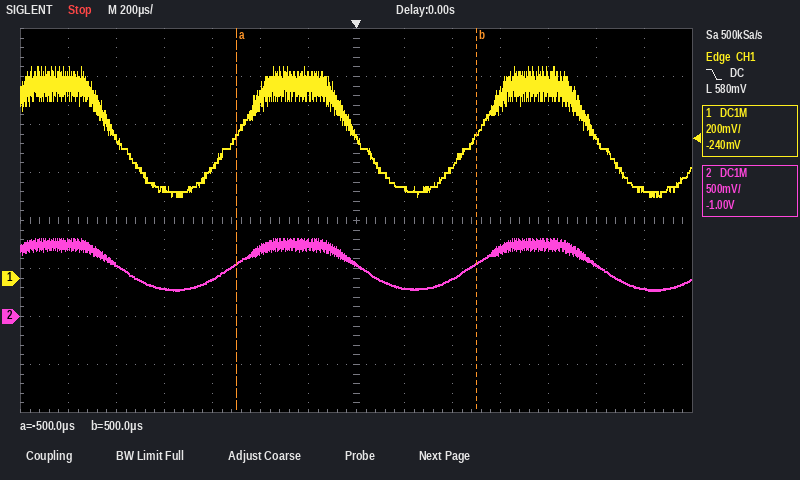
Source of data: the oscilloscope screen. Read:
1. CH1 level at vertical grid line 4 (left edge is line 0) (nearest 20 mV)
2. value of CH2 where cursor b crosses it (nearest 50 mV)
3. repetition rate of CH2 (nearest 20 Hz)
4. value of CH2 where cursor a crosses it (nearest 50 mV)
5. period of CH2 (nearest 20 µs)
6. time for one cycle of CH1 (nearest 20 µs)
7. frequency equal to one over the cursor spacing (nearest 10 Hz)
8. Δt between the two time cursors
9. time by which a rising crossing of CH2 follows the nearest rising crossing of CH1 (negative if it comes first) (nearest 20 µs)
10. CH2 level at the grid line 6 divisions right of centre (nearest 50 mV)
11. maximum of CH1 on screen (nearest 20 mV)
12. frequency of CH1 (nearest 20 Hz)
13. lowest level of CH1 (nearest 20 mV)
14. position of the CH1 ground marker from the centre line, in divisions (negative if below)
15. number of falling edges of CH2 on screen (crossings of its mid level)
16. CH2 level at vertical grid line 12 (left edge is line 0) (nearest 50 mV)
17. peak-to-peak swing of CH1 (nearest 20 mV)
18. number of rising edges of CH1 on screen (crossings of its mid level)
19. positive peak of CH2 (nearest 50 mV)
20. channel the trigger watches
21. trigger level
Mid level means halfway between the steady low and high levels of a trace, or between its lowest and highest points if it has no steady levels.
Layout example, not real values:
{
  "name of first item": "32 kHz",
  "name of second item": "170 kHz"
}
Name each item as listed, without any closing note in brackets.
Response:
{
  "CH1 level at vertical grid line 4 (left edge is line 0)": "460 mV",
  "value of CH2 where cursor b crosses it": "550 mV",
  "repetition rate of CH2": "1.00 kHz",
  "value of CH2 where cursor a crosses it": "550 mV",
  "period of CH2": "1.00 ms",
  "time for one cycle of CH1": "1.00 ms",
  "frequency equal to one over the cursor spacing": "1.00 kHz",
  "Δt between the two time cursors": "1.00 ms",
  "time by which a rising crossing of CH2 follows the nearest rising crossing of CH1 (negative if it comes first)": "-20 µs",
  "CH2 level at the grid line 6 divisions right of centre": "300 mV",
  "maximum of CH1 on screen": "880 mV",
  "frequency of CH1": "1.00 kHz",
  "lowest level of CH1": "340 mV",
  "position of the CH1 ground marker from the centre line, in divisions": "-1.2 div",
  "number of falling edges of CH2 on screen": "3",
  "CH2 level at vertical grid line 12 (left edge is line 0)": "550 mV",
  "peak-to-peak swing of CH1": "540 mV",
  "number of rising edges of CH1 on screen": "2",
  "positive peak of CH2": "800 mV",
  "channel the trigger watches": "CH1",
  "trigger level": "580 mV"
}
